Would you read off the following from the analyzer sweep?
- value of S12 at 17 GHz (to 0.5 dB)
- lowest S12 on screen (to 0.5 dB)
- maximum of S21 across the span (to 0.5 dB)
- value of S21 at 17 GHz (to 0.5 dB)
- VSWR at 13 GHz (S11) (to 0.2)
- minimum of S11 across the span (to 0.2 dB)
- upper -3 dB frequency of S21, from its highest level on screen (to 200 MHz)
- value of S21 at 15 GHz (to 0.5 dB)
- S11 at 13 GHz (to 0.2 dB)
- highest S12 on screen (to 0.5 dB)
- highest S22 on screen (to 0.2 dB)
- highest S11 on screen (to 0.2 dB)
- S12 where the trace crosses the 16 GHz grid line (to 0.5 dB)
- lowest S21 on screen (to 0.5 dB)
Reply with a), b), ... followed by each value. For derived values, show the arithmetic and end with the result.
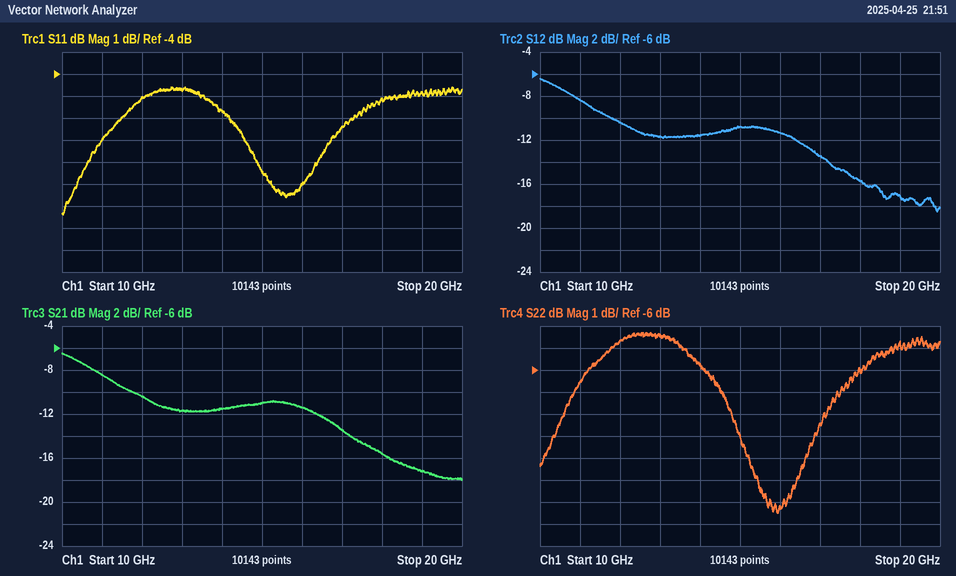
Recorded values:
a) -13.5 dB
b) -18.5 dB
c) -6.5 dB
d) -13.5 dB
e) |Γ| = 10^(-4.8/20) = 0.5754; VSWR = (1 + 0.5754)/(1 − 0.5754) ≈ 3.71, so 3.8 to the nearest 0.2
f) -10.4 dB
g) 11.4 GHz
h) -11.0 dB
i) -4.8 dB
j) -6.5 dB
k) -4.2 dB
l) -4.6 dB
m) -11.5 dB
n) -18.0 dB
